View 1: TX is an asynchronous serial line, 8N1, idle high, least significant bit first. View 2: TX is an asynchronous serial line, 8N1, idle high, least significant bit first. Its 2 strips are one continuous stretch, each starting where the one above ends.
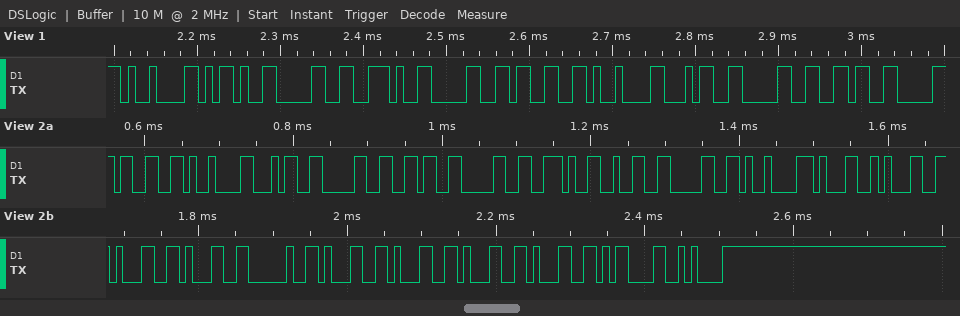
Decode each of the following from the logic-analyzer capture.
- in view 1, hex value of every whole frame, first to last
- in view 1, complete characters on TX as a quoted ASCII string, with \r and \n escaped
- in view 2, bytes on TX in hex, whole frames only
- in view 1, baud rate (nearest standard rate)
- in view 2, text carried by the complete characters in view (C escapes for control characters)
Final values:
0x09 0x2D 0x30 0x2E 0x30 0x33 0x09 0x34 0x30 0x36
"\t-0.03\t406"
33 09 34 30 36 30 2E 32 30 09 31 31 31 31 20 31 31 31 31 0D 0A
115200 baud
"3\t4060.20\t1111 1111\r\n"
